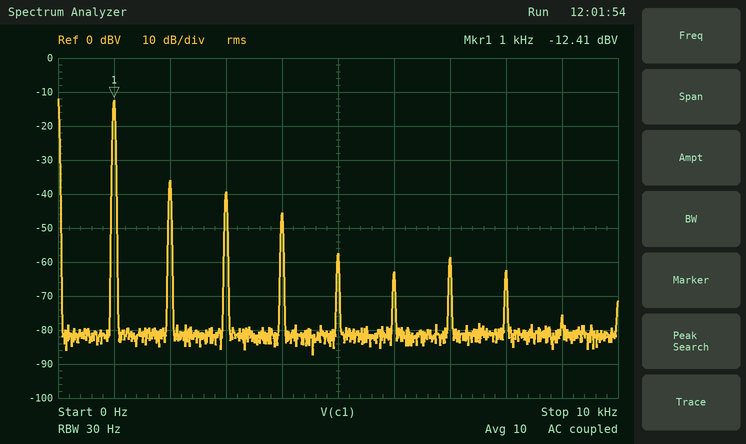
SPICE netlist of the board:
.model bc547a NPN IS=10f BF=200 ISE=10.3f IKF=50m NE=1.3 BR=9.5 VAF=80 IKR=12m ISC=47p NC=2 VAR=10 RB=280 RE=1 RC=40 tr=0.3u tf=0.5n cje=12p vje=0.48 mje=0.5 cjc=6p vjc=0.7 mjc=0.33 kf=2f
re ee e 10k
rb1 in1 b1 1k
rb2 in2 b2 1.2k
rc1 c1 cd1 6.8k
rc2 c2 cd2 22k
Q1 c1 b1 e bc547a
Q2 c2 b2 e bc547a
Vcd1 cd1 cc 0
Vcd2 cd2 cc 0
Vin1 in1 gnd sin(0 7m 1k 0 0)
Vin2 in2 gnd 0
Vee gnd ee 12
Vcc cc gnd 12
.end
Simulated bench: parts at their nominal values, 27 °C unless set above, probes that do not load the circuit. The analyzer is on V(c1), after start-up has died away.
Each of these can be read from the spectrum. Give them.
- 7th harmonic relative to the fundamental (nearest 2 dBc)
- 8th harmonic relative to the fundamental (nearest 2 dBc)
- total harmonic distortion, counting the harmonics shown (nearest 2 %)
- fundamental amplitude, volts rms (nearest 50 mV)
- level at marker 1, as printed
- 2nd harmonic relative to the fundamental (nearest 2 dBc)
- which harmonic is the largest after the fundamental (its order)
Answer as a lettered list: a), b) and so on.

a) -46 dBc
b) -50 dBc
c) 8 %
d) 250 mV
e) -12.41 dBV
f) -24 dBc
g) 2
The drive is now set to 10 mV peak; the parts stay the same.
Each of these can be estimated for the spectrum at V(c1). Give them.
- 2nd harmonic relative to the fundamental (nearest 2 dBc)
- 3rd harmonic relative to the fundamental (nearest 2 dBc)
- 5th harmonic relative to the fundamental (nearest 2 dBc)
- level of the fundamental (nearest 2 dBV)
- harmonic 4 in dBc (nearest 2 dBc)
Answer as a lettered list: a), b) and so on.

a) -18 dBc
b) -24 dBc
c) -38 dBc
d) -10 dBV
e) -38 dBc
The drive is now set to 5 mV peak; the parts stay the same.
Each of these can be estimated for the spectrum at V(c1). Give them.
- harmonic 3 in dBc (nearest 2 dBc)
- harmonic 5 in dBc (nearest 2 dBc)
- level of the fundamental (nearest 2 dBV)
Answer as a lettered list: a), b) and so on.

a) -40 dBc
b) -46 dBc
c) -14 dBV
